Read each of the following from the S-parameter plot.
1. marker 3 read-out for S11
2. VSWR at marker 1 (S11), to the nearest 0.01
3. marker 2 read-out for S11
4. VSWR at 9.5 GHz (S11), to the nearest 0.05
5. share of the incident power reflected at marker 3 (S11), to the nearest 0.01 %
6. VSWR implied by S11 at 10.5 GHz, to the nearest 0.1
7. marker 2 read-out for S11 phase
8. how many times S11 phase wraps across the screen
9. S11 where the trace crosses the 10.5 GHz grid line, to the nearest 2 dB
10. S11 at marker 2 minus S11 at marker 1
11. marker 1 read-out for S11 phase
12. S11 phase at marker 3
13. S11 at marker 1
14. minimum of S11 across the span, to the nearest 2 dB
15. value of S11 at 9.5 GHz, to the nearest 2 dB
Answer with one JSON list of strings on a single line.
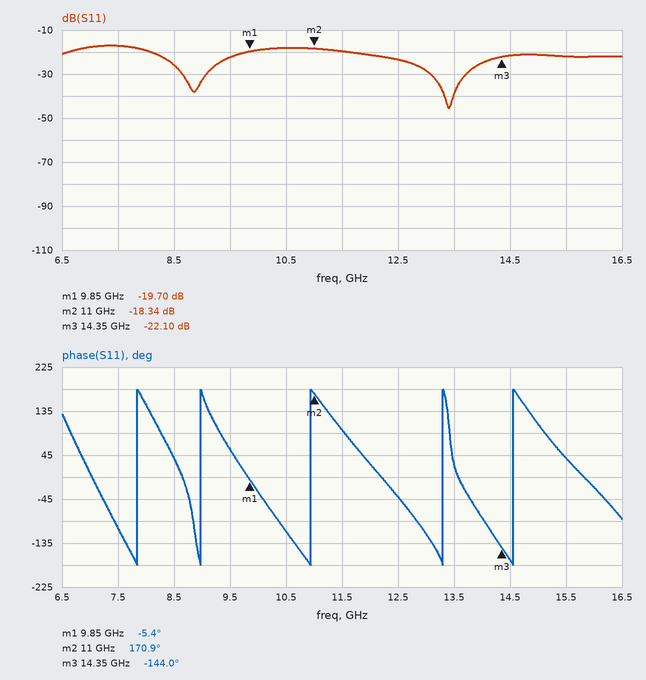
["-22.10 dB", "1.23", "-18.34 dB", "1.15", "0.62 %", "1.3", "170.9°", "5", "-18 dB", "1.36 dB", "-5.4°", "-144.0°", "-19.70 dB", "-46 dB", "-22 dB"]
